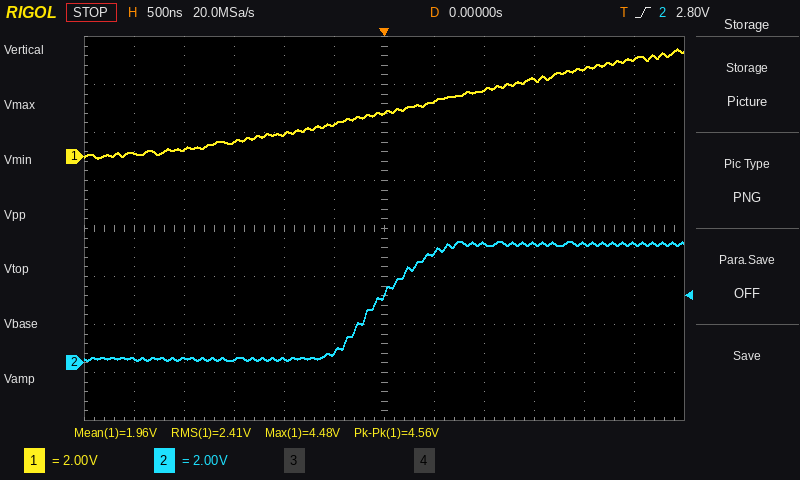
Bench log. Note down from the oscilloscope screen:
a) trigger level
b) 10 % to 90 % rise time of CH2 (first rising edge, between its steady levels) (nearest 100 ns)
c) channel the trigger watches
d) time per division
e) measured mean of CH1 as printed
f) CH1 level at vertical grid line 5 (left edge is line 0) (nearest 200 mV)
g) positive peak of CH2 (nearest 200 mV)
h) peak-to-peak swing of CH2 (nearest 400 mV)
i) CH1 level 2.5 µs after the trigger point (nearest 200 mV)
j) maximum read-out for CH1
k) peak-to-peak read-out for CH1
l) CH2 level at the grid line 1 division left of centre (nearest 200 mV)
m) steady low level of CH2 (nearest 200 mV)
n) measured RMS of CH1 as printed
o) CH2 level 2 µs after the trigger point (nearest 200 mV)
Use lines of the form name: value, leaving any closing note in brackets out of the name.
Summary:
trigger level: 2.80 V
10 % to 90 % rise time of CH2 (first rising edge, between its steady levels): 800 ns
channel the trigger watches: CH2
time per division: 500 ns
measured mean of CH1 as printed: 1.96 V
CH1 level at vertical grid line 5 (left edge is line 0): 1.4 V
positive peak of CH2: 5.0 V
peak-to-peak swing of CH2: 4.8 V
CH1 level 2.5 µs after the trigger point: 4.0 V
maximum read-out for CH1: 4.48 V
peak-to-peak read-out for CH1: 4.56 V
CH2 level at the grid line 1 division left of centre: 400 mV
steady low level of CH2: 200 mV
measured RMS of CH1 as printed: 2.41 V
CH2 level 2 µs after the trigger point: 5.0 V
